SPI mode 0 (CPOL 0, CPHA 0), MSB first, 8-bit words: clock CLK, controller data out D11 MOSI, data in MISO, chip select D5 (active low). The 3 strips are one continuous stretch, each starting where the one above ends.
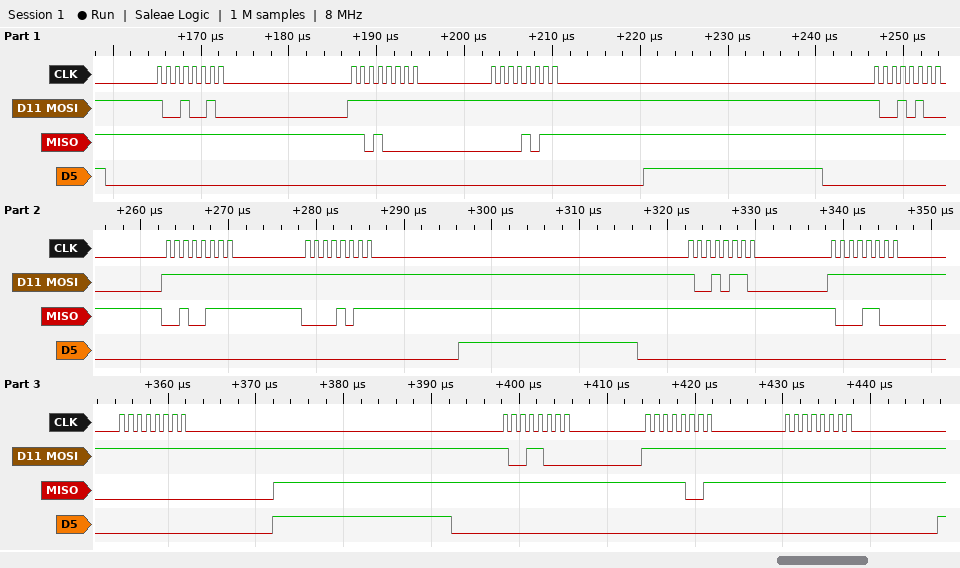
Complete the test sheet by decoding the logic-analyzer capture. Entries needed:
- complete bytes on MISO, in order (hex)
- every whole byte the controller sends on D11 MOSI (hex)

FF D0 0B FF 27 0B FF 8C 00 FF F9 FF
92 FF FF 94 FF FF 96 FF FF 98 FF FF
